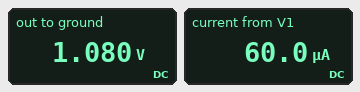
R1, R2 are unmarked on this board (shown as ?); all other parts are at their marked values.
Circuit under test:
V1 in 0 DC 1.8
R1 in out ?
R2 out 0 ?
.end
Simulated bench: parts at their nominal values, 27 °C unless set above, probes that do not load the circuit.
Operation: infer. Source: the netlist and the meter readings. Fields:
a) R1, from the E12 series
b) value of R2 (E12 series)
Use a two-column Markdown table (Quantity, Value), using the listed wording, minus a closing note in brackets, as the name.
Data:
| Quantity | Value |
|---|---|
| R1, from the E12 series | 12 kΩ |
| value of R2 | 18 kΩ |
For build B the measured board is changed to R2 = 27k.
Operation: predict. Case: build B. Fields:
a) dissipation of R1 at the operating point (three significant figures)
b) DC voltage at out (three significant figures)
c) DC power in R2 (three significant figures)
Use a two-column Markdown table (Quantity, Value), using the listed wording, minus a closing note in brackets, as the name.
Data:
| Quantity | Value |
|---|---|
| dissipation of R1 at the operating point | 25.6 µW |
| DC voltage at out | 1.25 V |
| DC power in R2 | 57.5 µW |
